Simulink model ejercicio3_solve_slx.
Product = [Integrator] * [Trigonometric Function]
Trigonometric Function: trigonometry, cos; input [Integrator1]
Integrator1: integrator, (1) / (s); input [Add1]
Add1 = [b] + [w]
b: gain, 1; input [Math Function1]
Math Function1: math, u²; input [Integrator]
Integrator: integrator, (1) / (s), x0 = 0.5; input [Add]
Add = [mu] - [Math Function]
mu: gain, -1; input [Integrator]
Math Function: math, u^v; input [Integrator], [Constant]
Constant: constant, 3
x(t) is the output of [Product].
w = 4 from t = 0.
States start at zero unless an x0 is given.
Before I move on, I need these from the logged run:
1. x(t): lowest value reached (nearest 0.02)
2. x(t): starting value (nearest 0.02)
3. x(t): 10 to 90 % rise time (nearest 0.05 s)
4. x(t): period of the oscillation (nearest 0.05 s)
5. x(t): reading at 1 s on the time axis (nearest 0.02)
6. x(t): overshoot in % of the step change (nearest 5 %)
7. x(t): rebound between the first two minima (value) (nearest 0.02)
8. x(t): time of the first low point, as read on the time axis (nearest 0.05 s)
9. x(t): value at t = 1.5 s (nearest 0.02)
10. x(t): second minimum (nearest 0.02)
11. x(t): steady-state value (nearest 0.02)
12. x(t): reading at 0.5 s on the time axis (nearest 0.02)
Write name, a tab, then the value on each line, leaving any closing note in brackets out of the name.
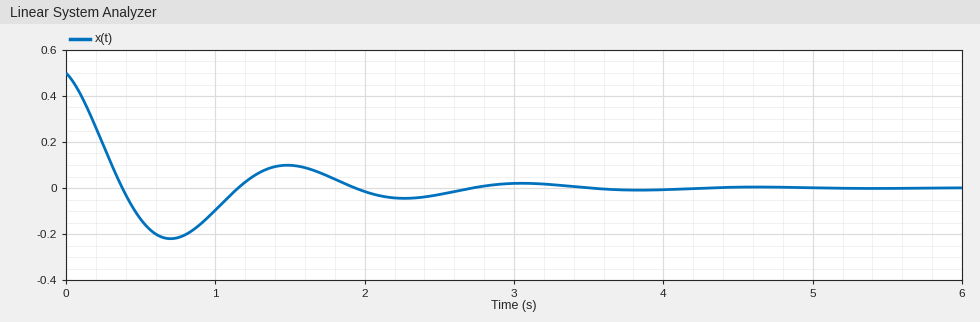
x(t): lowest value reached	-0.22
x(t): starting value	0.50
x(t): 10 to 90 % rise time	0.30 s
x(t): period of the oscillation	1.55 s
x(t): reading at 1 s on the time axis	-0.10
x(t): overshoot in % of the step change	45 %
x(t): rebound between the first two minima (value)	0.10
x(t): time of the first low point, as read on the time axis	0.70 s
x(t): value at t = 1.5 s	0.10
x(t): second minimum	-0.04
x(t): steady-state value	0.00
x(t): reading at 0.5 s on the time axis	-0.14
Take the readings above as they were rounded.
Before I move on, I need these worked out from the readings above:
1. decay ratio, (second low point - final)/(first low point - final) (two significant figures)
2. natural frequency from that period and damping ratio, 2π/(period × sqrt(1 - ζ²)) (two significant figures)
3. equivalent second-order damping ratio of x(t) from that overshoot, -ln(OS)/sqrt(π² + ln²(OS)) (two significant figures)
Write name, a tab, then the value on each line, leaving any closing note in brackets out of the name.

decay ratio, (second low point - final)/(first low point - final)	0.18
natural frequency from that period and damping ratio, 2π/(period × sqrt(1 - ζ²))	4.2 rad/s
equivalent second-order damping ratio of x(t) from that overshoot, -ln(OS)/sqrt(π² + ln²(OS))	0.25
